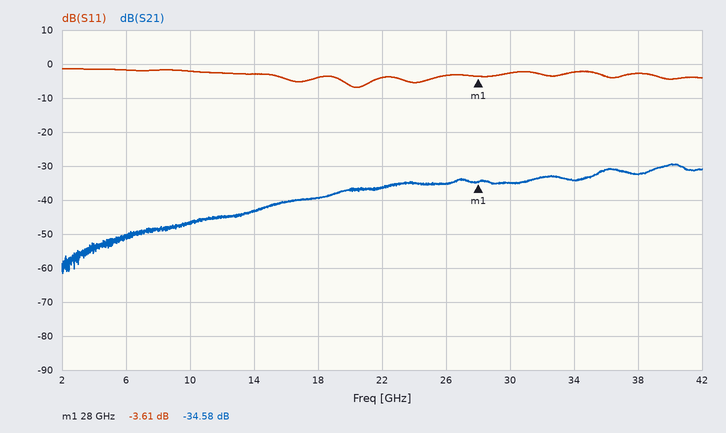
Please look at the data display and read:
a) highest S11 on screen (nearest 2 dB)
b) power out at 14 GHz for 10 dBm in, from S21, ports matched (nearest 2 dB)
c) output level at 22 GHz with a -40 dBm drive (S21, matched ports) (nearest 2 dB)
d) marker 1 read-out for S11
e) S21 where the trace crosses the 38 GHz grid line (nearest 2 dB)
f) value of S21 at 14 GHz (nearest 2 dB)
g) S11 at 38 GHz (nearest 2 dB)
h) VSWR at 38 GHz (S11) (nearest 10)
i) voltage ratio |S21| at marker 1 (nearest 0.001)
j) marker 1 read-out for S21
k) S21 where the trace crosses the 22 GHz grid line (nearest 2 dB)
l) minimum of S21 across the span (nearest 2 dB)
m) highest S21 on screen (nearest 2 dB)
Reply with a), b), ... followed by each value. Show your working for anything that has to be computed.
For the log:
a) -2 dB
b) 10 dBm + (-44 dB) = -34 dBm
c) -40 dBm + (-36 dB) = -76 dBm
d) -3.61 dB
e) -32 dB
f) -44 dB
g) -2 dB
h) |Γ| = 10^(-2/20) = 0.7943; VSWR = (1 + 0.7943)/(1 − 0.7943) ≈ 8.72, so 10 to the nearest 10
i) 10^(-34.58/20) ≈ 0.019
j) -34.58 dB
k) -36 dB
l) -62 dB
m) -30 dB
